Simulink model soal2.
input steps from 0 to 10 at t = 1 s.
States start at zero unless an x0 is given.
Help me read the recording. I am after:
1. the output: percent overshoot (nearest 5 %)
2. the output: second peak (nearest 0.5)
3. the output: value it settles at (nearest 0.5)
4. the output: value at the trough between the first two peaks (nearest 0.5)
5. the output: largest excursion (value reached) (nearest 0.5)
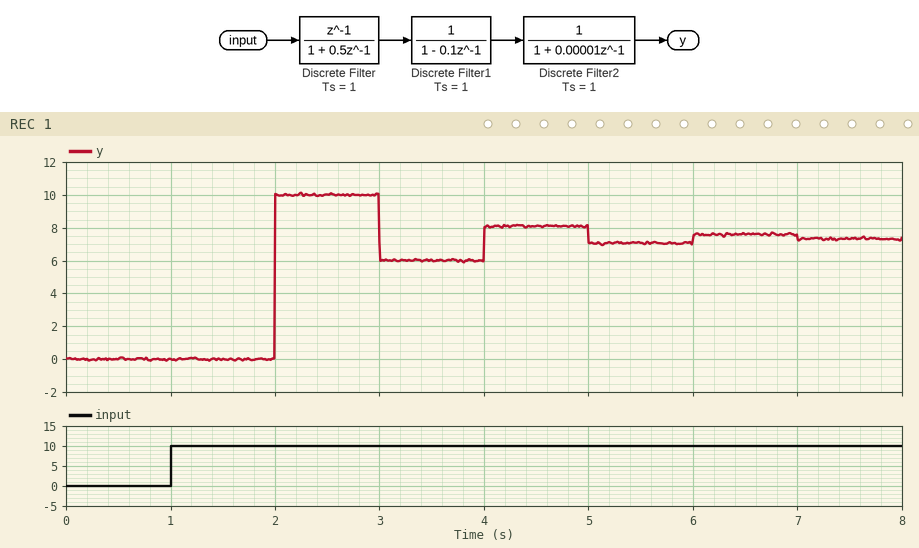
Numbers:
35 %
8.0
7.5
6.0
10.0
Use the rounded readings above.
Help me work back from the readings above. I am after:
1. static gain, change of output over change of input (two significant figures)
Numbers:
0.75
